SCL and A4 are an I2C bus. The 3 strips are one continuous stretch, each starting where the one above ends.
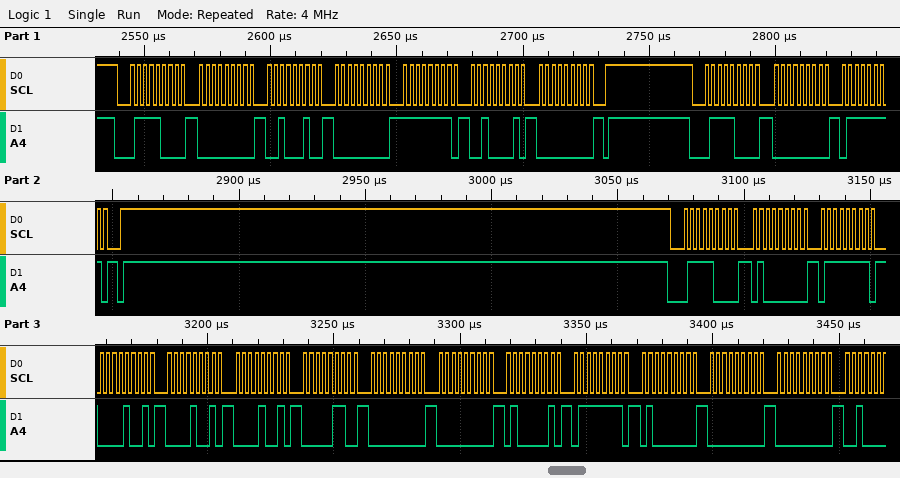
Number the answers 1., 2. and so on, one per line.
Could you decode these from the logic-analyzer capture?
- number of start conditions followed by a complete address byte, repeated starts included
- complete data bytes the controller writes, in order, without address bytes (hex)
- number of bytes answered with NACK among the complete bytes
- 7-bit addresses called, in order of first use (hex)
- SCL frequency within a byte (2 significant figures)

1. 3
2. 00 22 00 FF 21 00 00 7F 40 7F 09 09 09 06 00 00 41 7F 40 00 00
3. 0
4. 0x3C
5. 400 kHz
